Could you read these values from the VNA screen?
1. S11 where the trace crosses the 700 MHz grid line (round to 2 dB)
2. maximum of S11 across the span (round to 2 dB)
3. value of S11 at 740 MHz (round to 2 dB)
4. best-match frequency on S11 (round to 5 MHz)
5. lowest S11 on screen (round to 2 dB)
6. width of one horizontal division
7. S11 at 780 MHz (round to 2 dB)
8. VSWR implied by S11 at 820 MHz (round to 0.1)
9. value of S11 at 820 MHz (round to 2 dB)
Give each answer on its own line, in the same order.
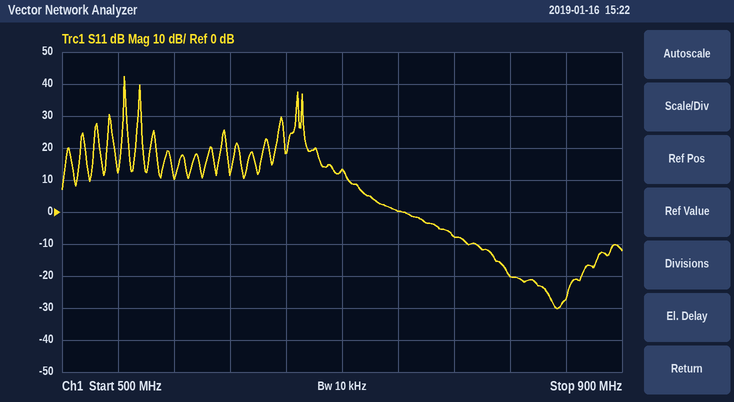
14 dB
42 dB
0 dB
855 MHz
-30 dB
40 MHz
-8 dB
1.2
-20 dB
